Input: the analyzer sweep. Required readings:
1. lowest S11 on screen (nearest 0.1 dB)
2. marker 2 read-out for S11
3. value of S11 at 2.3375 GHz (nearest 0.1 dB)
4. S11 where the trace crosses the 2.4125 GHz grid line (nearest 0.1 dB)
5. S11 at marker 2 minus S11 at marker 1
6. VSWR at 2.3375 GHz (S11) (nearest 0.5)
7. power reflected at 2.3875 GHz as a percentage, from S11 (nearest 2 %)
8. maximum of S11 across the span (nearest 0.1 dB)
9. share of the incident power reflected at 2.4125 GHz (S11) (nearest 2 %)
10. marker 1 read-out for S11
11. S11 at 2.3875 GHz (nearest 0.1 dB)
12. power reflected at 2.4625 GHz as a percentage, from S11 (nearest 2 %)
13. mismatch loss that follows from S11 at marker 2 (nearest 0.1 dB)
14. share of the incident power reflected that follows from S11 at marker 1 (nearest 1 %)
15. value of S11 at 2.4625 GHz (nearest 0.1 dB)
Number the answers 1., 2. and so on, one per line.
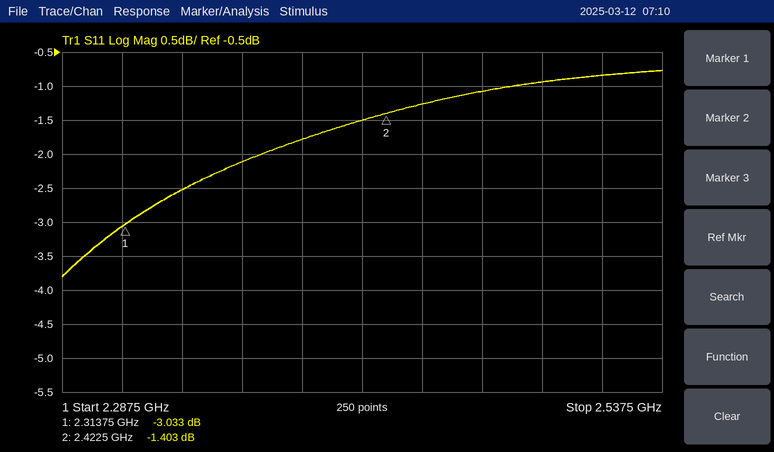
1. -3.8 dB
2. -1.403 dB
3. -2.5 dB
4. -1.5 dB
5. 1.630 dB
6. 7.0
7. 66 %
8. -0.8 dB
9. 70 %
10. -3.033 dB
11. -1.8 dB
12. 78 %
13. 5.6 dB
14. 50 %
15. -1.1 dB
